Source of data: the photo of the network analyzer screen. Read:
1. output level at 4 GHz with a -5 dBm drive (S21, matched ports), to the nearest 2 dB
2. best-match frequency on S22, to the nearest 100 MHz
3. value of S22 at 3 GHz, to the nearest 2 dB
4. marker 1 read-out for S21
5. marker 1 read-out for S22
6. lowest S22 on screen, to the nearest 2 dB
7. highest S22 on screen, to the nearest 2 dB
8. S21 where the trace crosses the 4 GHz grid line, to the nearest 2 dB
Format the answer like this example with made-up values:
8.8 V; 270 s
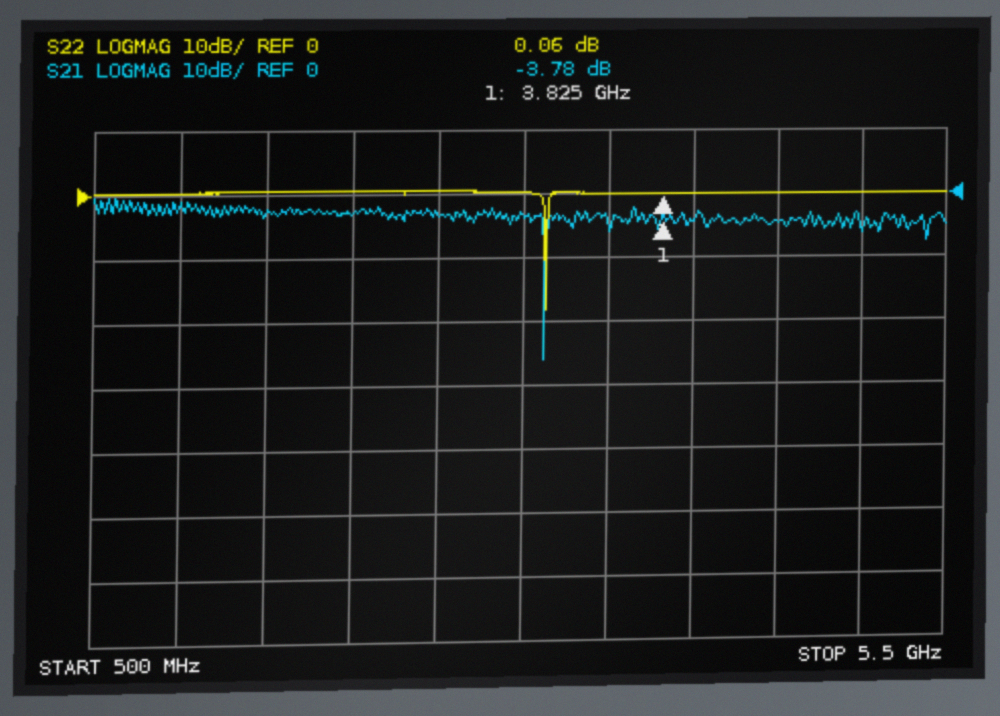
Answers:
-10 dBm; 3.1 GHz; 0 dB; -3.78 dB; 0.06 dB; -18 dB; 0 dB; -4 dB
